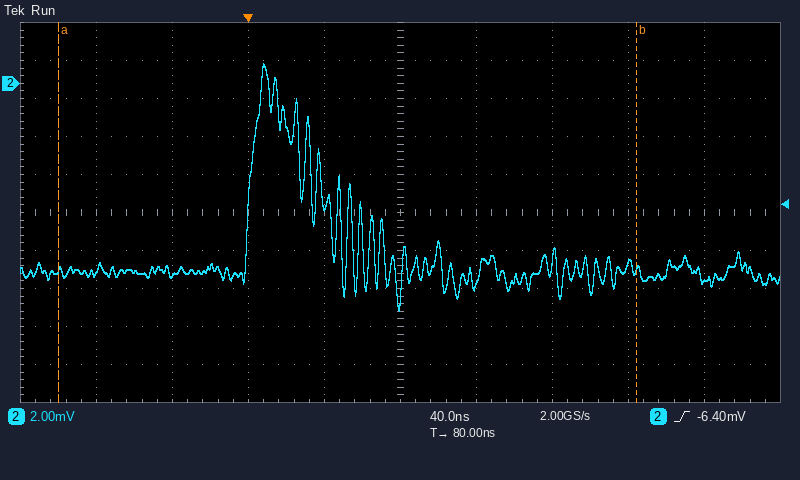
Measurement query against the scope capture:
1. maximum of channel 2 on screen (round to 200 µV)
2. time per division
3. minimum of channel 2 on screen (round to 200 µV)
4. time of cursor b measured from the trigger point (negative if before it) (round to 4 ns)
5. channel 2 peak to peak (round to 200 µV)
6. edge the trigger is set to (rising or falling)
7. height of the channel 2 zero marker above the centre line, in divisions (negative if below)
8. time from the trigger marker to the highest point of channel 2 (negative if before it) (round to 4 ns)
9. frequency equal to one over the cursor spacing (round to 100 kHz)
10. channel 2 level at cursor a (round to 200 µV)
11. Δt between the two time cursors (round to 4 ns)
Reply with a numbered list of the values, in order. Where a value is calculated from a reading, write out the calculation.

1. 1.0 mV
2. 40 ns
3. -12.0 mV
4. +204 ns
5. 1.0 mV − (-12.0 mV) = 13.0 mV
6. rising
7. +3.4 div
8. +8 ns
9. 1 / 304 ns ≈ 3.3 MHz
10. -9.8 mV
11. 304 ns
